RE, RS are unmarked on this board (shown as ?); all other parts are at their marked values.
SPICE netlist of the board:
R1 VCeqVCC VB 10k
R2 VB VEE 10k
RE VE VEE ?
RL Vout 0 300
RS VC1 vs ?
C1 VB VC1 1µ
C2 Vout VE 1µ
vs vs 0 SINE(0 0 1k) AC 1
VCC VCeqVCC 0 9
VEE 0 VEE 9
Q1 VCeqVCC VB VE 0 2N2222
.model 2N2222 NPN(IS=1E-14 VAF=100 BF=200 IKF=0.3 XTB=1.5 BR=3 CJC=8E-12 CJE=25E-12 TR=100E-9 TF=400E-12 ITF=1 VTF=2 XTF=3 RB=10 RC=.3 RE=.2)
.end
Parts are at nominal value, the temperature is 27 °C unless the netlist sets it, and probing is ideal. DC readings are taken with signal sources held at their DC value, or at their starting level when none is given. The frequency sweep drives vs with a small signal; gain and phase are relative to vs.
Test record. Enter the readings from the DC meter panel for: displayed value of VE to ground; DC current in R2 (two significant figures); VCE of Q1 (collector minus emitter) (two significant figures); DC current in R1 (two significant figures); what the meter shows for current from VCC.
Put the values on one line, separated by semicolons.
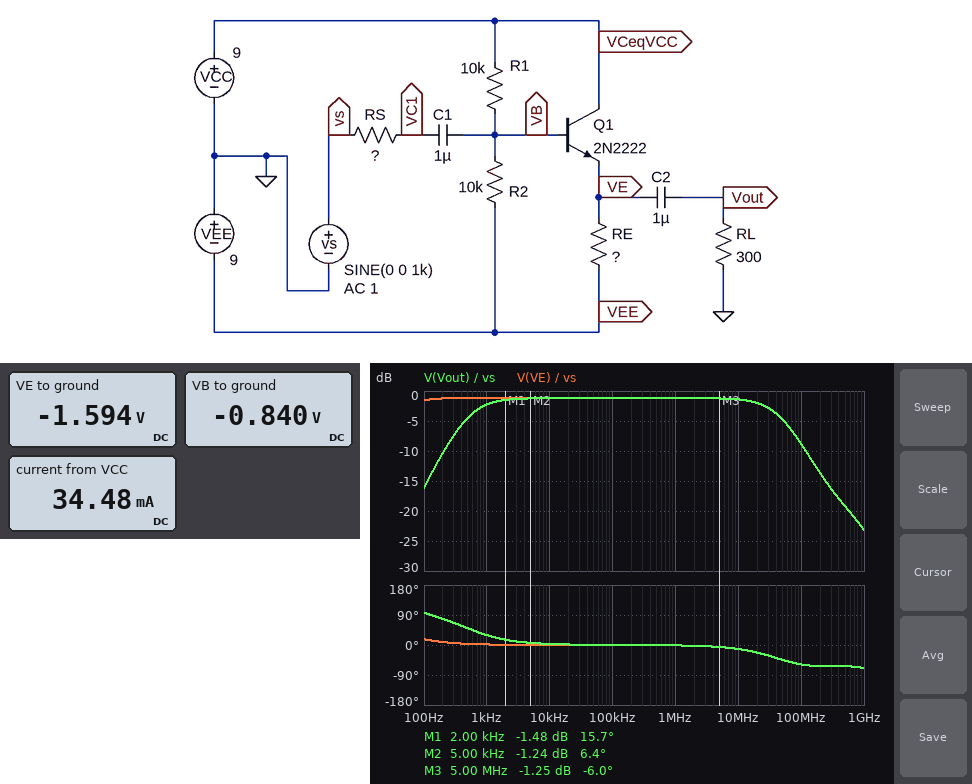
-1.594 V; 820 µA; 11 V; 980 µA; 34.48 mA
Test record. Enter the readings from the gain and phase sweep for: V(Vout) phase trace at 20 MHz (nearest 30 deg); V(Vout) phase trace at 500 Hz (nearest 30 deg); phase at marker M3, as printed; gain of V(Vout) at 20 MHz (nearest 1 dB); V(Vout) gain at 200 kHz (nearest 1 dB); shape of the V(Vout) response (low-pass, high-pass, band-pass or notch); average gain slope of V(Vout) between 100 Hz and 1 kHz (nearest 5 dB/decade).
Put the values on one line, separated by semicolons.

-30 deg; 60 deg; -6.0 deg; -2 dB; -1 dB; band-pass; 15 dB/decade
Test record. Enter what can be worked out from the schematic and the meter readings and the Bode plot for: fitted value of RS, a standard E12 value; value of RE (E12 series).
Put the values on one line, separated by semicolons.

560 Ω; 220 Ω
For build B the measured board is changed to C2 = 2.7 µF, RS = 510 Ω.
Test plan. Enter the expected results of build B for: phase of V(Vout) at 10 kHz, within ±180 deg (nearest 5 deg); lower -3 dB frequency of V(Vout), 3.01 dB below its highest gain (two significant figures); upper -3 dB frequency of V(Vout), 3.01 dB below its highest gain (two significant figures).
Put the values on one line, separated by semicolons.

0 deg; 200 Hz; 48 MHz
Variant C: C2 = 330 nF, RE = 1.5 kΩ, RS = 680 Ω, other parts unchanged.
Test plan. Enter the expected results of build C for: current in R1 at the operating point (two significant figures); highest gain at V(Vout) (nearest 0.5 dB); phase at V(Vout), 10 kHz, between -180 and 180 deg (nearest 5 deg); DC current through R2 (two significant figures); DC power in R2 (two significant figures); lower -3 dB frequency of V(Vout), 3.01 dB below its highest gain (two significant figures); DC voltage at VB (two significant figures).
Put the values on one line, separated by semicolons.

910 µA; -1.5 dB; 10 deg; 890 µA; 7.9 mW; 1.6 kHz; -130 mV
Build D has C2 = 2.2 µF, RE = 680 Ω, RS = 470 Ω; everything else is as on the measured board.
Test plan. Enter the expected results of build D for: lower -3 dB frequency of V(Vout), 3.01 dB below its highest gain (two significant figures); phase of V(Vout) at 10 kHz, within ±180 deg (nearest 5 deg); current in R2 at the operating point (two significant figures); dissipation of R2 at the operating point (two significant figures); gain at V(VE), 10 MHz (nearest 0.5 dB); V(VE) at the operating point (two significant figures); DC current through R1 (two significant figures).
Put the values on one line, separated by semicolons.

240 Hz; 0 deg; 870 µA; 7.6 mW; -1.0 dB; -1.0 V; 930 µA
